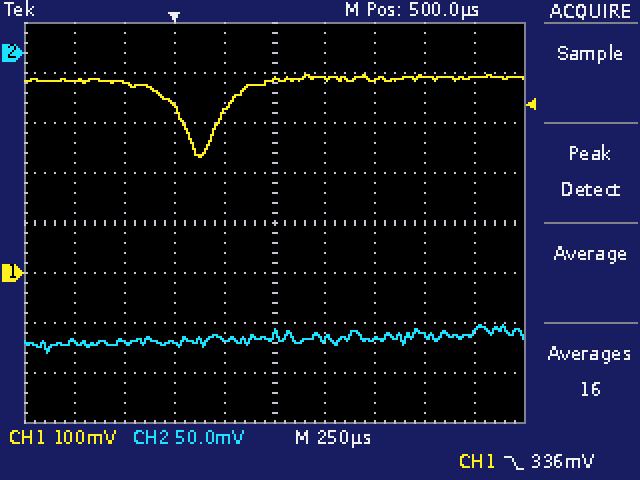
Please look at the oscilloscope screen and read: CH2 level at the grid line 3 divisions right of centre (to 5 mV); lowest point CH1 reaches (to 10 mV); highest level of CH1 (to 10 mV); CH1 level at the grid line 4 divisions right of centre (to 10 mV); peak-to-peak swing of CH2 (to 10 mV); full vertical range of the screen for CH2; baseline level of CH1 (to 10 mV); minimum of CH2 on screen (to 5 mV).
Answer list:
-285 mV
230 mV
400 mV
390 mV
30 mV
400 mV
390 mV
-300 mV
